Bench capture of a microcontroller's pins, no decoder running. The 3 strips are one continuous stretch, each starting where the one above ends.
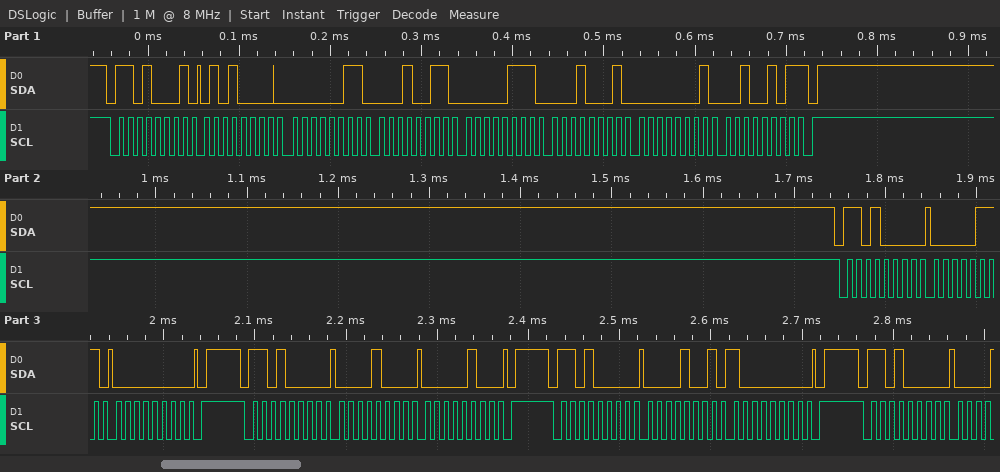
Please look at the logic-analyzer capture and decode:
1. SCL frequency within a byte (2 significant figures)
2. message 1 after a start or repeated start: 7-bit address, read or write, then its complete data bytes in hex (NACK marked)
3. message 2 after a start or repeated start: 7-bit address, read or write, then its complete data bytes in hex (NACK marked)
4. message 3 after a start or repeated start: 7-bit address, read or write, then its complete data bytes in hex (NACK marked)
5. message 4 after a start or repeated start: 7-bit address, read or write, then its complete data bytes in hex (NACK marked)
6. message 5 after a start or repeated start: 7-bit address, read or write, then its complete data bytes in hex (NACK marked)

100 kHz
0x68 read: 50 03 13 07 11 01 25 NACK
0x68 write: 07 00
0x68 write: 08 04
0x68 write: 09 80
0x68 write
